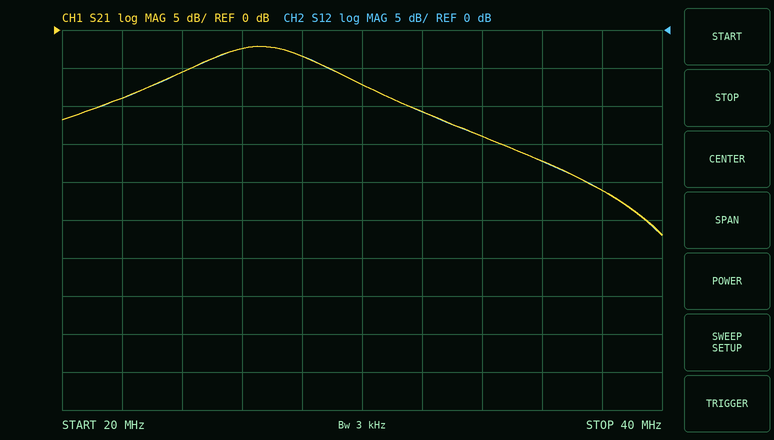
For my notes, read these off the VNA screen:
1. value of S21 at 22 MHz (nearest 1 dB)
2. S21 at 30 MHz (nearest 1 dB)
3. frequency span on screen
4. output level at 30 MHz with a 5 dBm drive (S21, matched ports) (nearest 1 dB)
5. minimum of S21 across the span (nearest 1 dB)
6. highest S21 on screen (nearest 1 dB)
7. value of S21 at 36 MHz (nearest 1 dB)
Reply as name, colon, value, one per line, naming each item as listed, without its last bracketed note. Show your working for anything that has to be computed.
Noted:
value of S21 at 22 MHz: -9 dB
S21 at 30 MHz: -7 dB
frequency span on screen: 20 MHz
output level at 30 MHz with a 5 dBm drive (S21, matched ports): 5 dBm + (-7 dB) = -2 dBm
minimum of S21 across the span: -27 dB
highest S21 on screen: -2 dB
value of S21 at 36 MHz: -17 dB
